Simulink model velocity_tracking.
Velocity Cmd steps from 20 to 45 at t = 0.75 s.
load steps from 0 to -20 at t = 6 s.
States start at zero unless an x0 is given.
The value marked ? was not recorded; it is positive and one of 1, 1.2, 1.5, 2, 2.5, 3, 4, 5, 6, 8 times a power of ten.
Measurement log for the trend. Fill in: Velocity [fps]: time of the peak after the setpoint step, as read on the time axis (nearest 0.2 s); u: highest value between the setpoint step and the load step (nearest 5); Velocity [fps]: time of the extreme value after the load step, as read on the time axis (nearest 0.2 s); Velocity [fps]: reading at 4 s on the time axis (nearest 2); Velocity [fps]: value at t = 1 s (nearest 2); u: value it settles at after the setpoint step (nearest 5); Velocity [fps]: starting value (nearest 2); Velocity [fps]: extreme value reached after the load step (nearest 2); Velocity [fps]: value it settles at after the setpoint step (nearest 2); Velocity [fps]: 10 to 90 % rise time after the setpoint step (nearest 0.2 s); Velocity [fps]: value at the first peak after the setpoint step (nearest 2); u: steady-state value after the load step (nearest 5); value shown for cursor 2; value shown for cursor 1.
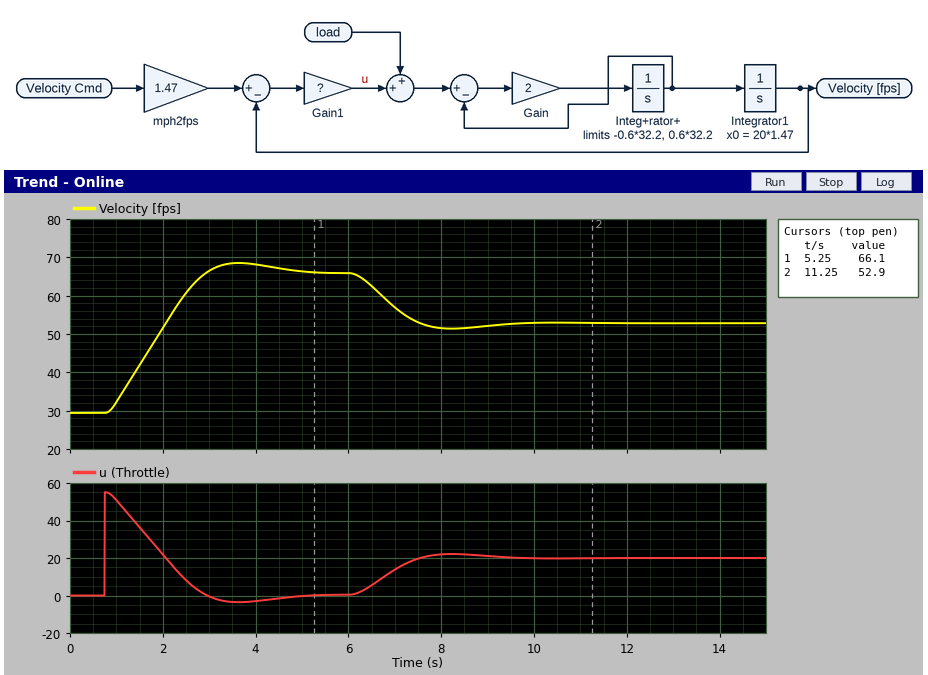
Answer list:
3.6 s
55
8.2 s
68
32
0
30
52
66
1.6 s
68
20
52.9
66.1
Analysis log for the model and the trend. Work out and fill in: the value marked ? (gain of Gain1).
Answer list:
1.5
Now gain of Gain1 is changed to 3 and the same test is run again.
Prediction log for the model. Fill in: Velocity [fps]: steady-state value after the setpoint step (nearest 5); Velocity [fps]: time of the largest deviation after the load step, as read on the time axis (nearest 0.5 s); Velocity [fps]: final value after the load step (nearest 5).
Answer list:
65
7.5 s
60
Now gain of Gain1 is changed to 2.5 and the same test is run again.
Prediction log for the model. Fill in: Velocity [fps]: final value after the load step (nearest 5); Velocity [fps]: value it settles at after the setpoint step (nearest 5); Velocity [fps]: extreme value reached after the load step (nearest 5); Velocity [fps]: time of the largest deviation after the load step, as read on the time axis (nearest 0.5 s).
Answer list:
60
65
55
7.5 s
